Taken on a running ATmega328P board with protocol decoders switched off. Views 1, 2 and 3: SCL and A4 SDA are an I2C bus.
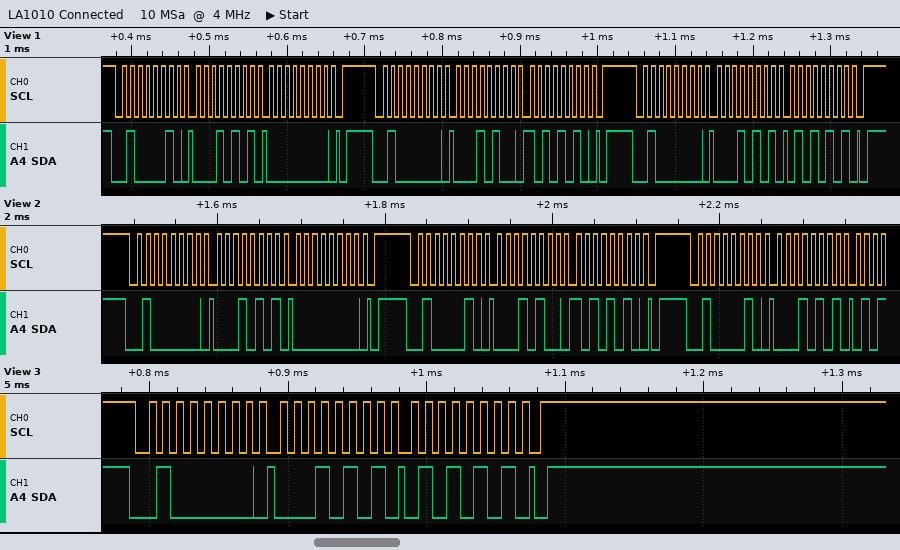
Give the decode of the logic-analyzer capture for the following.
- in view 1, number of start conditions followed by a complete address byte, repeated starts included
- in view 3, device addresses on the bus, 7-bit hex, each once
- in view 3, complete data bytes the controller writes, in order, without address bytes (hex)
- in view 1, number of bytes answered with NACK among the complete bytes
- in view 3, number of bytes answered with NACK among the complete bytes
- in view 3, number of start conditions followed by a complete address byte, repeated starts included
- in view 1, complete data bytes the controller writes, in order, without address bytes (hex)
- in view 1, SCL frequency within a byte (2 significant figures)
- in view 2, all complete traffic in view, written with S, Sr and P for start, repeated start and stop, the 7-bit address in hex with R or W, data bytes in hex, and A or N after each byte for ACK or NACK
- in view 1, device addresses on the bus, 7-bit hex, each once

3
0x20
15 55
0
0
1
15 00 14 AA 15 55
100 kHz
S 20W A 15 A 00 A P S 21W A 14 A AA A P S 21W A 15 A
0x21 0x20
